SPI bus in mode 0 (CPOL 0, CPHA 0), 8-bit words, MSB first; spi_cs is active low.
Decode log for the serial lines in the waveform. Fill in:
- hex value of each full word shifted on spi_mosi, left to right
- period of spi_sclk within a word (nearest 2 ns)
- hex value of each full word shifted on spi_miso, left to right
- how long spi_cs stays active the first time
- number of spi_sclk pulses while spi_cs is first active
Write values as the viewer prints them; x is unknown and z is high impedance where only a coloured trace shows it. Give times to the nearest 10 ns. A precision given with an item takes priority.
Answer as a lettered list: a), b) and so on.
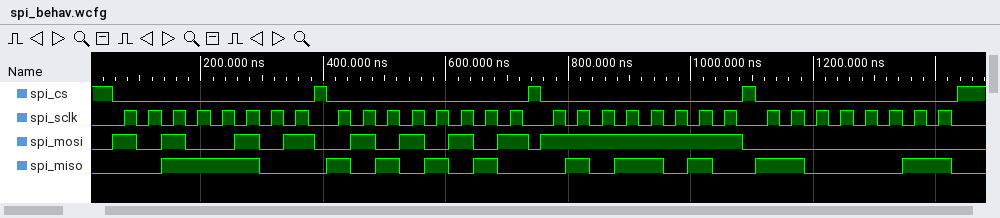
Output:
a) A5, 55, FF, 00
b) 40 ns
c) 3C, AA, 5A, C3
d) 330 ns
e) 8
